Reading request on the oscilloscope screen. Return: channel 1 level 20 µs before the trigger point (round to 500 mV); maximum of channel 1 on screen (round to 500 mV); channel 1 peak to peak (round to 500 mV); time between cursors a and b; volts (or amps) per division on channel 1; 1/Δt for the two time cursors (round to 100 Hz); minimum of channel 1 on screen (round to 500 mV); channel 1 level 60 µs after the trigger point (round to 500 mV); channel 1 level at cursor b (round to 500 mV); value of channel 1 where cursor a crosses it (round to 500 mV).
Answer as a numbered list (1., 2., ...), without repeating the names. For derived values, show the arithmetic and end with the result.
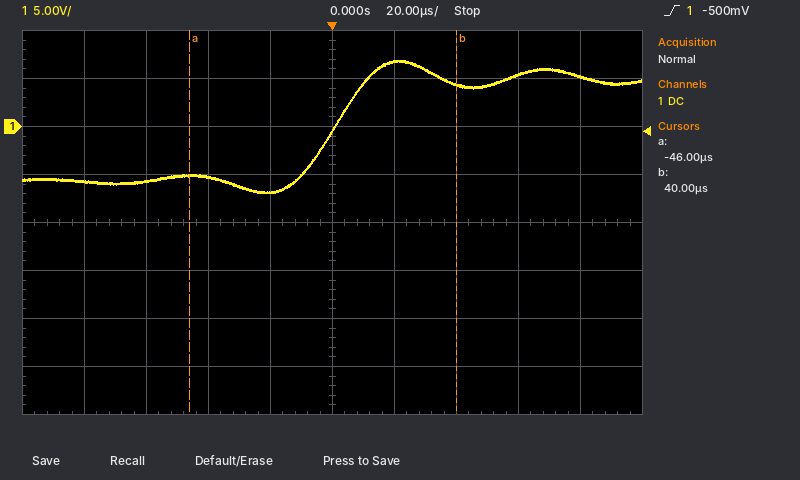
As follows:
1. -7.0 V
2. 7.0 V
3. 7.0 V − (-7.0 V) = 14.0 V
4. 40 µs − (-46 µs) = 86 µs
5. 5 V
6. 1 / 86 µs ≈ 11.6 kHz
7. -7.0 V
8. 5.5 V
9. 4.5 V
10. -5.0 V
